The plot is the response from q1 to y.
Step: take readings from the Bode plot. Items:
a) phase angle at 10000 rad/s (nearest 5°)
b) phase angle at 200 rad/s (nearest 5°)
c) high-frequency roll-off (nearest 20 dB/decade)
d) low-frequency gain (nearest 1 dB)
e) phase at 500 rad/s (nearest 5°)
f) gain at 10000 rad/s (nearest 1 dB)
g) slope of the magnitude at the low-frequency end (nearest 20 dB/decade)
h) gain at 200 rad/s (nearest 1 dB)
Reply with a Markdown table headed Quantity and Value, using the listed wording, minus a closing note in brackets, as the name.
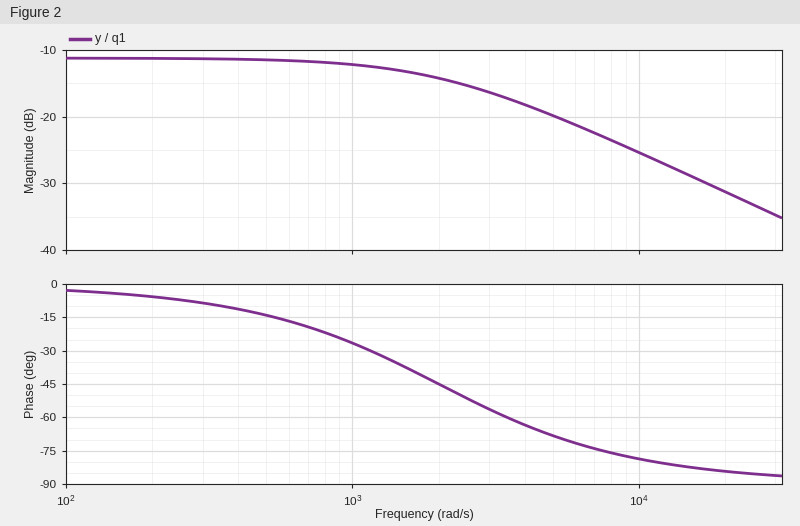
| Quantity | Value |
|---|---|
| phase angle at 10000 rad/s | -80° |
| phase angle at 200 rad/s | -5° |
| high-frequency roll-off | -20 dB/decade |
| low-frequency gain | -11 dB |
| phase at 500 rad/s | -15° |
| gain at 10000 rad/s | -25 dB |
| slope of the magnitude at the low-frequency end | 0 dB/decade |
| gain at 200 rad/s | -11 dB |
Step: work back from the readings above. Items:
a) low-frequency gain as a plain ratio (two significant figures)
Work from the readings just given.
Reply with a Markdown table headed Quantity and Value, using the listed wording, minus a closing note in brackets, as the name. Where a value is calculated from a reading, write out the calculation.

| Quantity | Value |
|---|---|
| low-frequency gain as a plain ratio | 10^(-11 / 20) = 0.28 |
